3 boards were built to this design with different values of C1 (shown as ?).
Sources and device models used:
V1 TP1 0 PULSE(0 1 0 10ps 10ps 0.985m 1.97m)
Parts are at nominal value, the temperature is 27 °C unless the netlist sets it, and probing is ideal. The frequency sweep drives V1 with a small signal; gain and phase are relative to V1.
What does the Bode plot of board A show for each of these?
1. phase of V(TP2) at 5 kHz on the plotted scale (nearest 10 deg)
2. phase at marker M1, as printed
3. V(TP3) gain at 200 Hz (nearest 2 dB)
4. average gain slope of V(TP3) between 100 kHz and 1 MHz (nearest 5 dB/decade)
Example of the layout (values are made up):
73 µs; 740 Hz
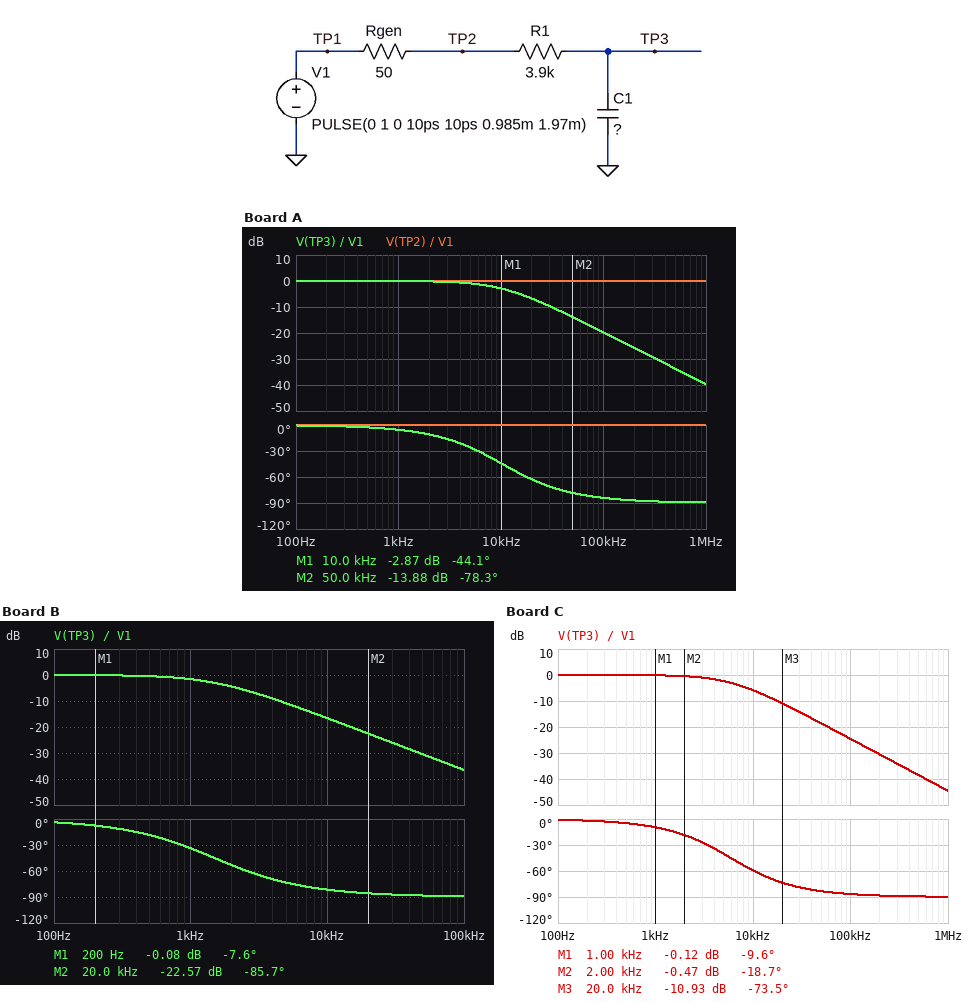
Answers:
0 deg; -44.1 deg; 0 dB; -20 dB/decade
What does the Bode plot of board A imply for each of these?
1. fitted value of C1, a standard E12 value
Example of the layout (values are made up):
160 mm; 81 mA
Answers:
3.9 nF
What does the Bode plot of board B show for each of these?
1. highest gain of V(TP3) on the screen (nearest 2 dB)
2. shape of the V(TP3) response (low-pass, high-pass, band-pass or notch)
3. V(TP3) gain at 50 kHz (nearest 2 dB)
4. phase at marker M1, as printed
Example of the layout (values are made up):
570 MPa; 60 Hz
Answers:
0 dB; low-pass; -30 dB; -7.6 deg
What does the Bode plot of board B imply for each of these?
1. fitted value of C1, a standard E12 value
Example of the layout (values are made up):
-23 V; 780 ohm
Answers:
27 nF
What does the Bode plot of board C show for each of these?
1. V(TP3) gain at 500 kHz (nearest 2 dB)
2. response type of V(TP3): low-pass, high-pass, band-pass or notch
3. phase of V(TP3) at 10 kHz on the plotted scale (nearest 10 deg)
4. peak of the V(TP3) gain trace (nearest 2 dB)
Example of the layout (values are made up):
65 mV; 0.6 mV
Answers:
-38 dB; low-pass; -60 deg; 0 dB
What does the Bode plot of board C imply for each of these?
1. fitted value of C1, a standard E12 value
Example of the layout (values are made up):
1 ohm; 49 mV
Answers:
6.8 nF
